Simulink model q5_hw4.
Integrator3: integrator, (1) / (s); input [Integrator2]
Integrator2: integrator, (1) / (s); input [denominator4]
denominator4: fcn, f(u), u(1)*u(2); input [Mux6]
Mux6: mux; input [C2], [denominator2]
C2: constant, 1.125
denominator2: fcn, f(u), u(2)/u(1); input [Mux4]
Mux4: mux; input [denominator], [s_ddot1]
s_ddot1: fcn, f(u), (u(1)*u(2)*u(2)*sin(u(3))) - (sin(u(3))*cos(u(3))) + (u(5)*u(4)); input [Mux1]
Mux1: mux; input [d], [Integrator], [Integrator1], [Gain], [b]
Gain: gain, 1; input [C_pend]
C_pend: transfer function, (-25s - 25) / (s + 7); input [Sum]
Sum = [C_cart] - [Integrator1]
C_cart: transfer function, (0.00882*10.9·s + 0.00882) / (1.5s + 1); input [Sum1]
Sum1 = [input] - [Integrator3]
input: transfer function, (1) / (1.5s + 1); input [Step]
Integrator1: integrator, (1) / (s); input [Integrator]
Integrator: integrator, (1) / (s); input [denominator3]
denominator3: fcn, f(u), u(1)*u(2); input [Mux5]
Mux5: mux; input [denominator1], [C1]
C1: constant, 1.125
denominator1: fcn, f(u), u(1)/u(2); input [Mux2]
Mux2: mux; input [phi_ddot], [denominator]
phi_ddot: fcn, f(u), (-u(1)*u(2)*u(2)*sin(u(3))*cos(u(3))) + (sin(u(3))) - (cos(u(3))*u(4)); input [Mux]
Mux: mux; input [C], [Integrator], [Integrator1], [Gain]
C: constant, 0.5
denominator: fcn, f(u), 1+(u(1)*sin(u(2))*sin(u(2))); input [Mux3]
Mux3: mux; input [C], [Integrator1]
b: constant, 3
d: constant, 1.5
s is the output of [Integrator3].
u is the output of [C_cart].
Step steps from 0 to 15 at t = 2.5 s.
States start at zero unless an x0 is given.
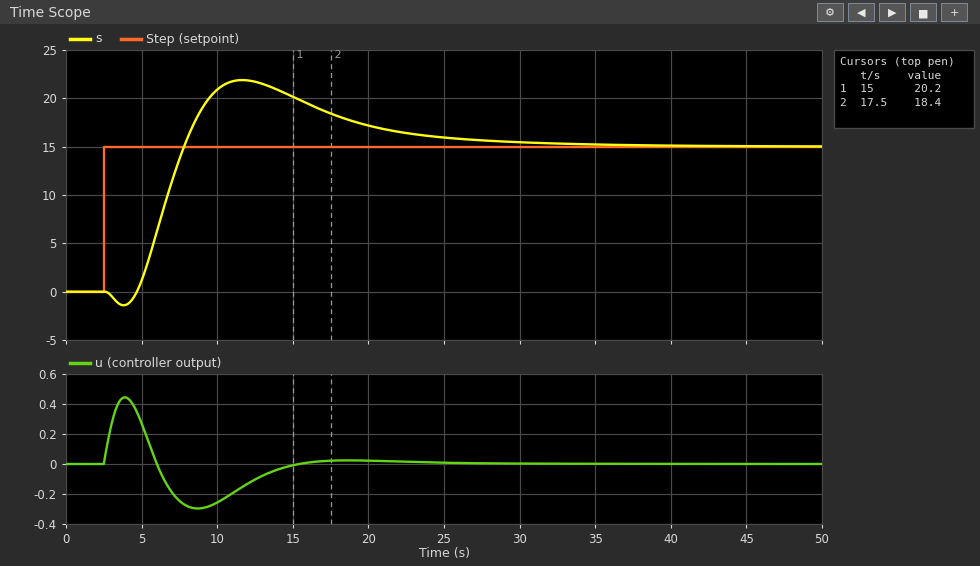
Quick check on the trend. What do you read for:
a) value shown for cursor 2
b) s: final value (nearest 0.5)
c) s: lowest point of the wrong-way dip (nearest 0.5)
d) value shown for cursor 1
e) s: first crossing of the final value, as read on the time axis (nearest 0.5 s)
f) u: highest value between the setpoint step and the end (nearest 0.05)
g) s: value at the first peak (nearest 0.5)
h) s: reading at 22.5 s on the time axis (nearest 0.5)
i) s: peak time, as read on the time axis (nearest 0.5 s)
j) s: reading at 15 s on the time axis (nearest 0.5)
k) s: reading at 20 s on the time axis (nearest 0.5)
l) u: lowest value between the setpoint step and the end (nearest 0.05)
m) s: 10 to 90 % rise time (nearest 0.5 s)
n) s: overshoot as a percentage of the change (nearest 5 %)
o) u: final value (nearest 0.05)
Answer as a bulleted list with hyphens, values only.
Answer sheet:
- 18.4
- 15.0
- -1.5
- 20.2
- 8.0 s
- 0.45
- 22.0
- 16.5
- 11.5 s
- 20.0
- 17.0
- -0.30
- 2.5 s
- 45 %
- 0.00
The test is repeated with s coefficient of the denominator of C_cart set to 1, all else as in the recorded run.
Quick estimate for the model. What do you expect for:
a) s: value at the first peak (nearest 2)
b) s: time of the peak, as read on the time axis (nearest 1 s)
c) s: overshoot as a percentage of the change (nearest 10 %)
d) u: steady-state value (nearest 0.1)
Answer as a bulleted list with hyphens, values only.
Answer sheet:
- 24
- 8 s
- 60 %
- 0.0
